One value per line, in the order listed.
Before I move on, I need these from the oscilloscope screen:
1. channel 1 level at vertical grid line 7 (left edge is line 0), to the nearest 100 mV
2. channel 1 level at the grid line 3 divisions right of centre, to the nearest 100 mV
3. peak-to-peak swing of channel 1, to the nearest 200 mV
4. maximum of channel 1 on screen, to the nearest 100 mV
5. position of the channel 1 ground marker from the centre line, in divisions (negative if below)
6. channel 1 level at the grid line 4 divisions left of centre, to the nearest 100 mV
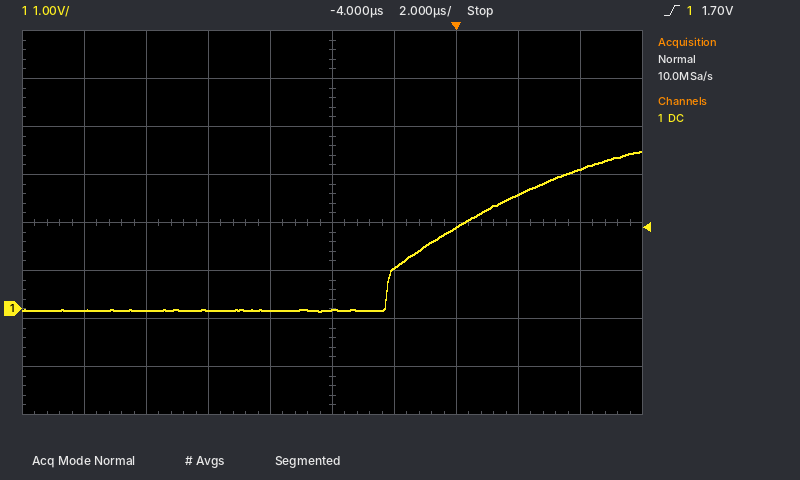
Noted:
1.7 V
2.4 V
3.4 V
3.3 V
-1.8 div
0.0 V
